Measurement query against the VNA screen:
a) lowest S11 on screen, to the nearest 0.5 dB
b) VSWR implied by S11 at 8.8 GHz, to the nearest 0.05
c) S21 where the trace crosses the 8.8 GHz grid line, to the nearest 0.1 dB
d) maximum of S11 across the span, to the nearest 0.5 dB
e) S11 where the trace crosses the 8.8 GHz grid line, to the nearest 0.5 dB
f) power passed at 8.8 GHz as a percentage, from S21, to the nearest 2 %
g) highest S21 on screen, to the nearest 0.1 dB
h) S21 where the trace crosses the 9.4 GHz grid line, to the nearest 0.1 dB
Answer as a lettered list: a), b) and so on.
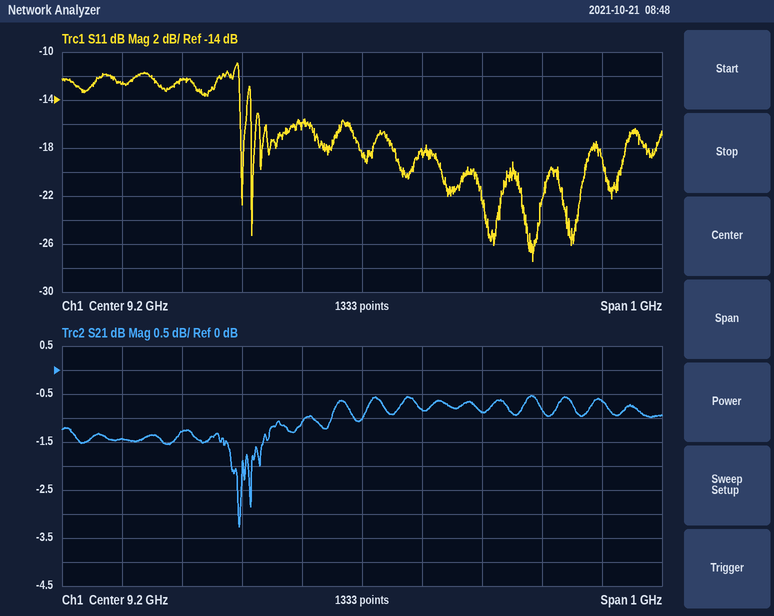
a) -27.5 dB
b) 1.60
c) -1.4 dB
d) -11.0 dB
e) -12.5 dB
f) 72 %
g) -0.5 dB
h) -0.9 dB
